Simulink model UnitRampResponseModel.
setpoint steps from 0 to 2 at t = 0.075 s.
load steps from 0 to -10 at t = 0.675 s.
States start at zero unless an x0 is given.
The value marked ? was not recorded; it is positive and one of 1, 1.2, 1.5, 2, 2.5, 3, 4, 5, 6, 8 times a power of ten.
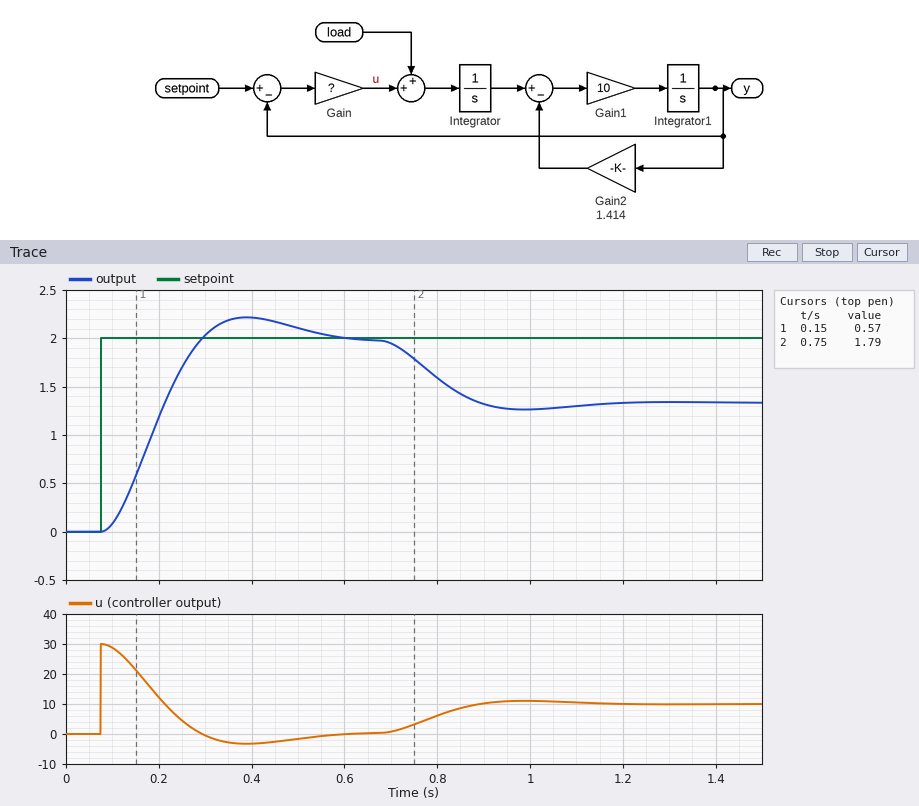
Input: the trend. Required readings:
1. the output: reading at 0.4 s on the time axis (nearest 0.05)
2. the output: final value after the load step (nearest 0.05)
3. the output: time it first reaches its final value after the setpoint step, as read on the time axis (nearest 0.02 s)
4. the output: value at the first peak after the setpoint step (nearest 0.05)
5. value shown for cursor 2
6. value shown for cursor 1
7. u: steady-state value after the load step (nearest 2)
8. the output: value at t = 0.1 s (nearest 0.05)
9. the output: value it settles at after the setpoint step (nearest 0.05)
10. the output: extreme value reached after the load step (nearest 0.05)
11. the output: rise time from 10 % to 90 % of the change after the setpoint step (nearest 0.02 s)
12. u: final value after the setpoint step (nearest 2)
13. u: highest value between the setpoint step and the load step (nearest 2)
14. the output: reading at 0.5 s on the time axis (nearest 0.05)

2.20
1.35
0.30 s
2.20
1.79
0.57
10
0.10
2.00
1.25
0.14 s
0
30
2.10
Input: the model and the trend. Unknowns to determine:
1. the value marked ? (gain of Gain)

15
